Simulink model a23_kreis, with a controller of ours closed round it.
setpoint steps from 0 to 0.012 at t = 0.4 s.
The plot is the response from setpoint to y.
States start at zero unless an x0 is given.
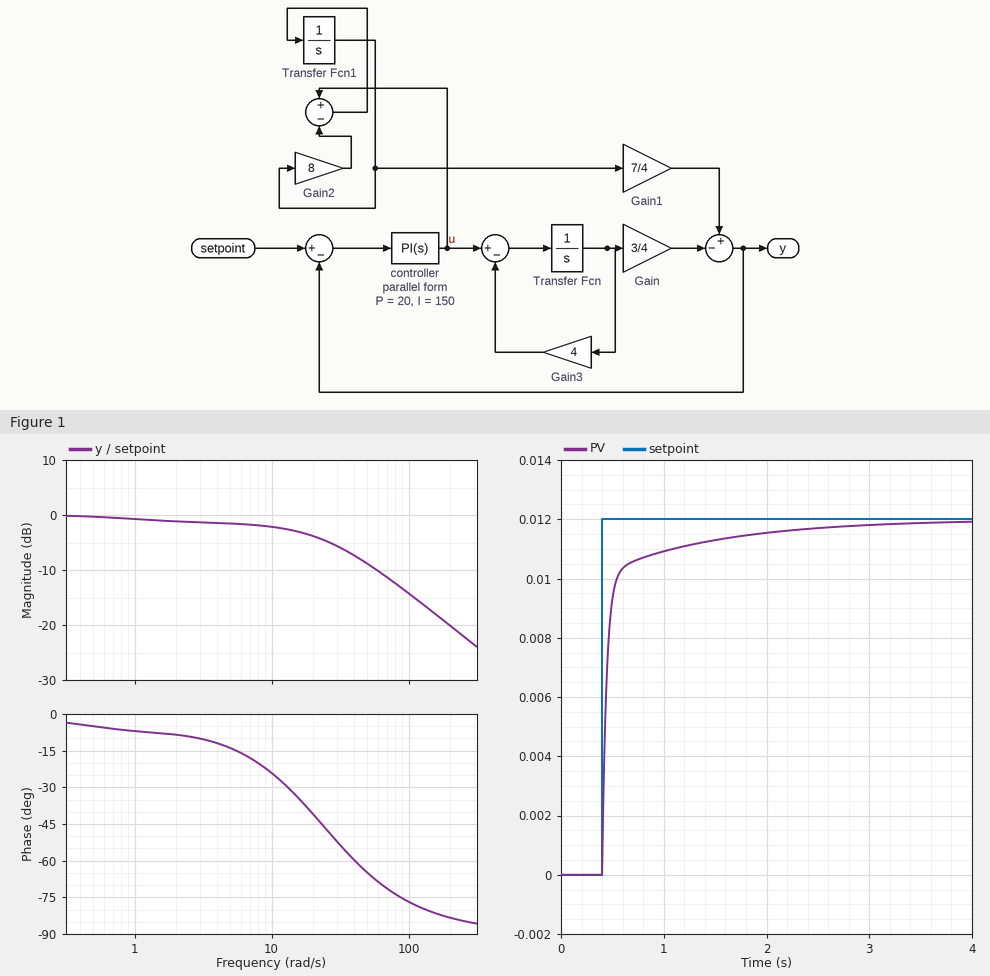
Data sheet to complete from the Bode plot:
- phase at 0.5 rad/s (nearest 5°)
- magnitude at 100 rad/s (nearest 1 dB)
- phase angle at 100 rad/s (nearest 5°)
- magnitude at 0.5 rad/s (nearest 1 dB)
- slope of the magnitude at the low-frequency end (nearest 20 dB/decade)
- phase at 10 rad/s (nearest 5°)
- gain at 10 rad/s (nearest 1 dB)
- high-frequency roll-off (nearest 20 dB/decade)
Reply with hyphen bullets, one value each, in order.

- -5°
- -14 dB
- -75°
- 0 dB
- 0 dB/decade
- -25°
- -2 dB
- -20 dB/decade
